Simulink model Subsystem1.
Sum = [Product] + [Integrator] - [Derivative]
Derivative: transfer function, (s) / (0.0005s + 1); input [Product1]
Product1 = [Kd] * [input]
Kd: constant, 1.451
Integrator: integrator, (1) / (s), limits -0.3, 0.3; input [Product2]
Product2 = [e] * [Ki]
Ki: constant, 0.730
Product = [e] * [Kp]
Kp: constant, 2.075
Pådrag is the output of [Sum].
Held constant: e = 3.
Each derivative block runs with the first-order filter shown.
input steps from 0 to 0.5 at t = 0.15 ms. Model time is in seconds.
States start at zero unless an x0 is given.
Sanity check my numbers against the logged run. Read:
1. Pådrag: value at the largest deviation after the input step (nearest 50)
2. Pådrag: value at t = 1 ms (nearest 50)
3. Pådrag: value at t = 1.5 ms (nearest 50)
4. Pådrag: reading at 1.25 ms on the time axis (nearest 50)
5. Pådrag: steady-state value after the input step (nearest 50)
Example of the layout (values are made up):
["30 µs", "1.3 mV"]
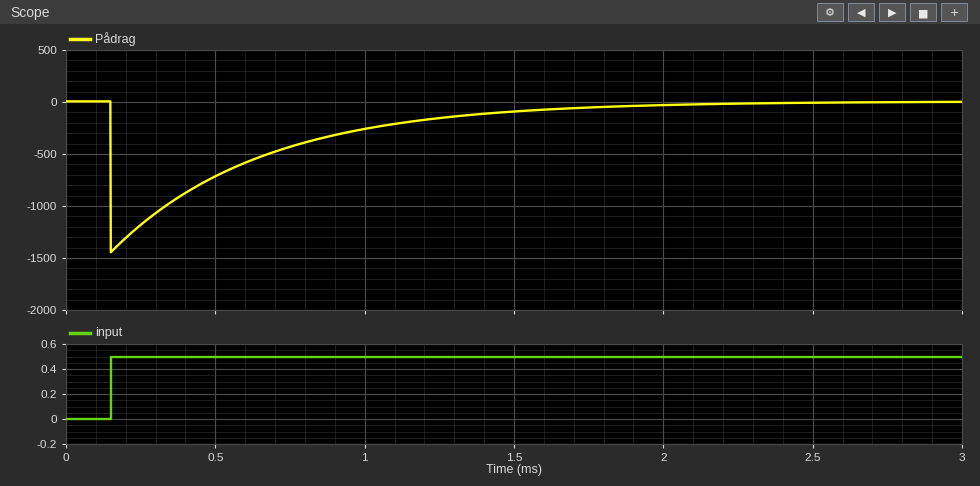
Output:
["-1450", "-250", "-100", "-150", "0"]
